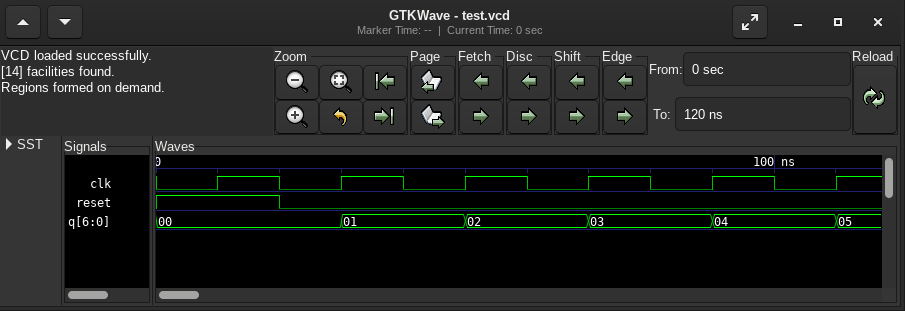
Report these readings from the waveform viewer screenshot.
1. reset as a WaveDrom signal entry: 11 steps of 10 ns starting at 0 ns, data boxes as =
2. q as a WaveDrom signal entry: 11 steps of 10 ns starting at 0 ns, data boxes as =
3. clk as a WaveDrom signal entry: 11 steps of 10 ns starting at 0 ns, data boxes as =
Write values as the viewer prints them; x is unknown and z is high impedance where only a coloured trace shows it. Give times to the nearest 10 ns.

{name: 'reset', wave: '1.0........'}
{name: 'q', wave: '=..=.=.=.=.', data: '00 01 02 03 04'}
{name: 'clk', wave: '01010101010'}
